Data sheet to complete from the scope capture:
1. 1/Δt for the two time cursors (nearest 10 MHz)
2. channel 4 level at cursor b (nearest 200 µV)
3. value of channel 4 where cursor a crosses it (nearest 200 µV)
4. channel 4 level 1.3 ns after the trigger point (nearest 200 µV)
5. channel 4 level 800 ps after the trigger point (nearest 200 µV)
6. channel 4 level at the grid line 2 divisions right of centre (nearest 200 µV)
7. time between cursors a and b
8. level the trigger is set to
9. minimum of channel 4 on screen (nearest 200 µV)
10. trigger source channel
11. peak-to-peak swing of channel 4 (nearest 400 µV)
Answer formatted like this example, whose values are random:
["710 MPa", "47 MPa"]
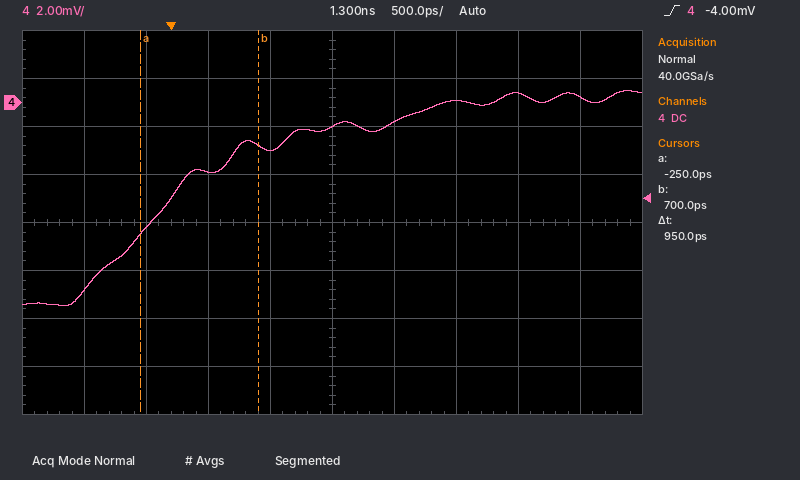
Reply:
["1.05 GHz", "-1.8 mV", "-5.4 mV", "-1.0 mV", "-2.0 mV", "0.0 mV", "950 ps", "-4.00 mV", "-8.4 mV", "channel 4", "8.8 mV"]
